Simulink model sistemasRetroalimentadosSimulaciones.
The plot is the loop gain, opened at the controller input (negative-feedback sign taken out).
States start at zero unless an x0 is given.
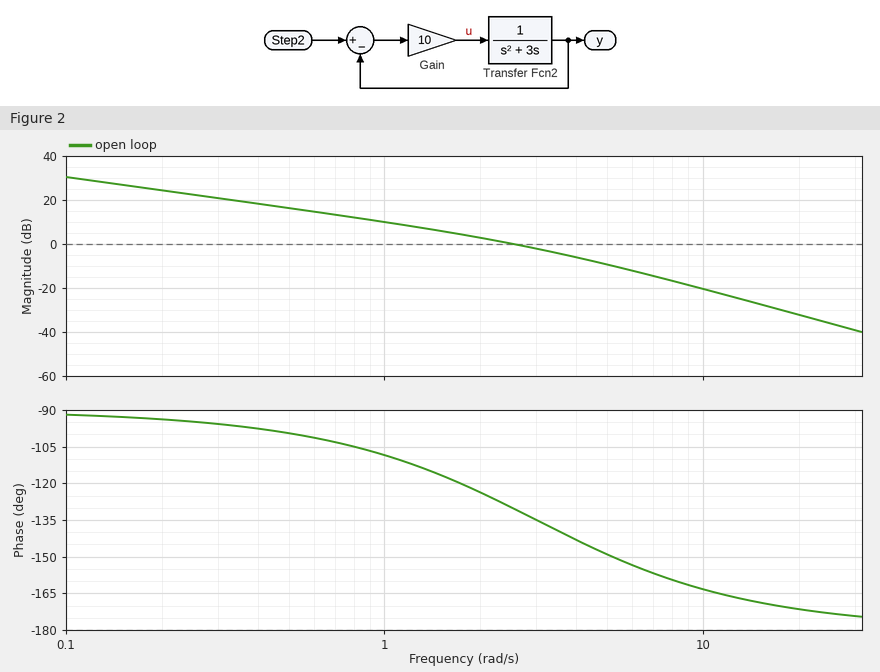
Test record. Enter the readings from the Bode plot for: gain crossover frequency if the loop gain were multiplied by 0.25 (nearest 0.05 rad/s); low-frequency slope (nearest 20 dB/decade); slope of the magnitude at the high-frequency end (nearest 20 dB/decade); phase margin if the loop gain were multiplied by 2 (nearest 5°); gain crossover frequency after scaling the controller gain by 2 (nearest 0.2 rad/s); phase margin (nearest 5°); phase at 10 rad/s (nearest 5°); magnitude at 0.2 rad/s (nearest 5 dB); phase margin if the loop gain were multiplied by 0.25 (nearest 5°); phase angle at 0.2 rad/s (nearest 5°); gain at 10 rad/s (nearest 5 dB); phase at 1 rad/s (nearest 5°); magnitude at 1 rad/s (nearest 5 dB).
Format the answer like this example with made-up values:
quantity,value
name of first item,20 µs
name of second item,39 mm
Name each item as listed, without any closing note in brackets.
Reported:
quantity,value
gain crossover frequency if the loop gain were multiplied by 0.25,0.80 rad/s
low-frequency slope,-20 dB/decade
slope of the magnitude at the high-frequency end,-40 dB/decade
phase margin if the loop gain were multiplied by 2,35°
gain crossover frequency after scaling the controller gain by 2,4.0 rad/s
phase margin,50°
phase at 10 rad/s,-165°
magnitude at 0.2 rad/s,25 dB
phase margin if the loop gain were multiplied by 0.25,75°
phase angle at 0.2 rad/s,-95°
gain at 10 rad/s,-20 dB
phase at 1 rad/s,-110°
magnitude at 1 rad/s,10 dB
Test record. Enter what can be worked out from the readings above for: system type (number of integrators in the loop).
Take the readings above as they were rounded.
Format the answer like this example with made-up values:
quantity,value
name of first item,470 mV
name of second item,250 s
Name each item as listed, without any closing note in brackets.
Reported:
quantity,value
system type,1
